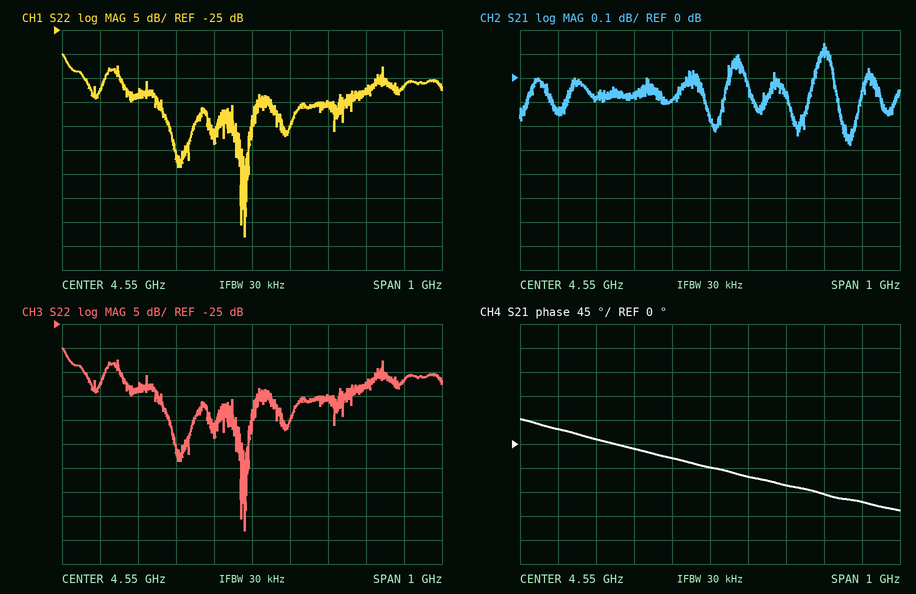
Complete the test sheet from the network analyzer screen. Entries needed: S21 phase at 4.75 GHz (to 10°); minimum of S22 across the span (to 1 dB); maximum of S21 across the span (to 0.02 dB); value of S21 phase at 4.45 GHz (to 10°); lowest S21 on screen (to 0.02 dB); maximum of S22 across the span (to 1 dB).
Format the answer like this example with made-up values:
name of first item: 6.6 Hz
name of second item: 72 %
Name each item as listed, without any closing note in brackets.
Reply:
S21 phase at 4.75 GHz: -80°
minimum of S22 across the span: -68 dB
maximum of S21 across the span: 0.14 dB
value of S21 phase at 4.45 GHz: -30°
lowest S21 on screen: -0.28 dB
maximum of S22 across the span: -30 dB
